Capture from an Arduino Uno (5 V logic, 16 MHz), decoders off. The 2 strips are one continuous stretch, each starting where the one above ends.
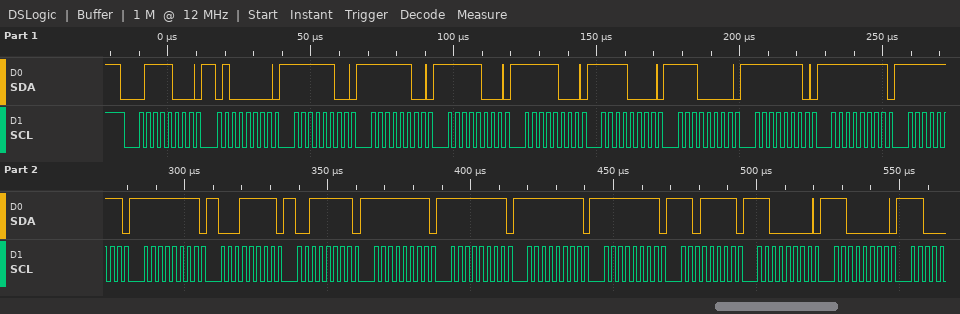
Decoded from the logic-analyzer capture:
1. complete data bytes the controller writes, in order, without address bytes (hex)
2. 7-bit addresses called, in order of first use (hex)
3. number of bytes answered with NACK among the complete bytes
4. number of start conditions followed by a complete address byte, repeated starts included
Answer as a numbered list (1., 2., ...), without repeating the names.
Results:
1. 40 FC FC F8 F8 F0 E0 FE FF FF FF 1F 3F FF FF FF FF DF C0 C0
2. 0x3C
3. 0
4. 1
